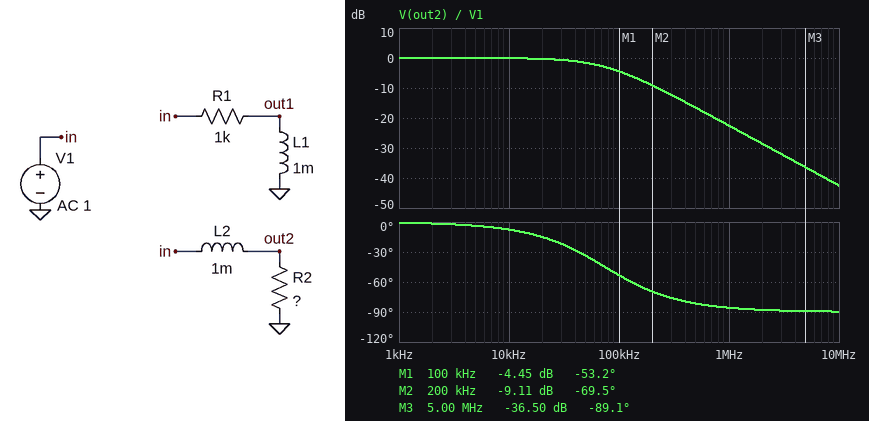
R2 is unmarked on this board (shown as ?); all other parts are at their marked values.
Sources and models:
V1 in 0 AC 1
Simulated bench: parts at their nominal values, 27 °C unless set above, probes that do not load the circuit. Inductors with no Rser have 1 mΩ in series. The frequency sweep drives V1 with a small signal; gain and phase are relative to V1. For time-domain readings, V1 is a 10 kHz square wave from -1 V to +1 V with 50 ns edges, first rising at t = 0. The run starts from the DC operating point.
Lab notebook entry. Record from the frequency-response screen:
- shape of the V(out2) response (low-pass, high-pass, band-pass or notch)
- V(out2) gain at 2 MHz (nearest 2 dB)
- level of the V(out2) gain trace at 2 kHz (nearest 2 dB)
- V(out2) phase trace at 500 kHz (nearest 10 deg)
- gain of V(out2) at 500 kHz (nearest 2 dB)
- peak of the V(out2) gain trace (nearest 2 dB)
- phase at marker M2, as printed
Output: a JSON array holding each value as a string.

["low-pass", "-28 dB", "0 dB", "-80 deg", "-16 dB", "0 dB", "-69.5 deg"]
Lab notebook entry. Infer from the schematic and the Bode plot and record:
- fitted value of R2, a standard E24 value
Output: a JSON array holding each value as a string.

["470 Ω"]
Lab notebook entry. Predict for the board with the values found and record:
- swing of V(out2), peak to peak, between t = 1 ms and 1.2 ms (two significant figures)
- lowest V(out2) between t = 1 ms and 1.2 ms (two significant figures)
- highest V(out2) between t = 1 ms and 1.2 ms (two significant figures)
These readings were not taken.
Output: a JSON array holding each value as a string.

["2.0 V", "-1.0 V", "1.0 V"]
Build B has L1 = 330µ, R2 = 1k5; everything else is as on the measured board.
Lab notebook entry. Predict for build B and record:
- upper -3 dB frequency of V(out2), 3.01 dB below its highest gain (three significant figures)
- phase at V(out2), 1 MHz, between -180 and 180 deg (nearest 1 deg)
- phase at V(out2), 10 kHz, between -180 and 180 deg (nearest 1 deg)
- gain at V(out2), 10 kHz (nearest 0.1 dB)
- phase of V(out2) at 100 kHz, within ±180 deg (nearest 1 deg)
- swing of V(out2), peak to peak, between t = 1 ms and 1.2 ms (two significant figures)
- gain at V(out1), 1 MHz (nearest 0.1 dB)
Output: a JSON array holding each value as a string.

["239 kHz", "-77 deg", "-2 deg", "0 dB", "-23 deg", "2.0 V", "-0.9 dB"]
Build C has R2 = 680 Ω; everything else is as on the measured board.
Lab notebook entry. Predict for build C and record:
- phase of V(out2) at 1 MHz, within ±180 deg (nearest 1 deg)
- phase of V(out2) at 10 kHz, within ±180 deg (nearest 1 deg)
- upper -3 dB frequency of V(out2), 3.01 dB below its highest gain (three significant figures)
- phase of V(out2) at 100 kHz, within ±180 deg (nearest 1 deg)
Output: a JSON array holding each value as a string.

["-84 deg", "-5 deg", "108 kHz", "-43 deg"]
